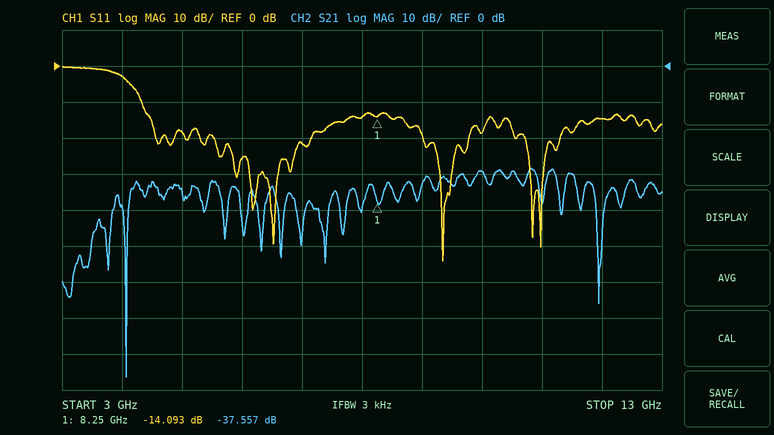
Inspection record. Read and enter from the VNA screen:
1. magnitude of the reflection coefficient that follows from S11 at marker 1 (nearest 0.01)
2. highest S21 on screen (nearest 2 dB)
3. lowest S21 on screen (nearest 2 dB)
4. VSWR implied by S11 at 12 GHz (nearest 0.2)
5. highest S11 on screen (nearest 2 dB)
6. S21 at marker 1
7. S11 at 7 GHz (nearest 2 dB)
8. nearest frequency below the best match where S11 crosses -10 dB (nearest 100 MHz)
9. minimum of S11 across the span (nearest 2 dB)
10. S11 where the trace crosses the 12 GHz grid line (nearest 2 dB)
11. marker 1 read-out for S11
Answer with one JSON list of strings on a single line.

["0.20", "-28 dB", "-86 dB", "1.4", "0 dB", "-37.557 dB", "-22 dB", "4.3 GHz", "-54 dB", "-14 dB", "-14.093 dB"]
